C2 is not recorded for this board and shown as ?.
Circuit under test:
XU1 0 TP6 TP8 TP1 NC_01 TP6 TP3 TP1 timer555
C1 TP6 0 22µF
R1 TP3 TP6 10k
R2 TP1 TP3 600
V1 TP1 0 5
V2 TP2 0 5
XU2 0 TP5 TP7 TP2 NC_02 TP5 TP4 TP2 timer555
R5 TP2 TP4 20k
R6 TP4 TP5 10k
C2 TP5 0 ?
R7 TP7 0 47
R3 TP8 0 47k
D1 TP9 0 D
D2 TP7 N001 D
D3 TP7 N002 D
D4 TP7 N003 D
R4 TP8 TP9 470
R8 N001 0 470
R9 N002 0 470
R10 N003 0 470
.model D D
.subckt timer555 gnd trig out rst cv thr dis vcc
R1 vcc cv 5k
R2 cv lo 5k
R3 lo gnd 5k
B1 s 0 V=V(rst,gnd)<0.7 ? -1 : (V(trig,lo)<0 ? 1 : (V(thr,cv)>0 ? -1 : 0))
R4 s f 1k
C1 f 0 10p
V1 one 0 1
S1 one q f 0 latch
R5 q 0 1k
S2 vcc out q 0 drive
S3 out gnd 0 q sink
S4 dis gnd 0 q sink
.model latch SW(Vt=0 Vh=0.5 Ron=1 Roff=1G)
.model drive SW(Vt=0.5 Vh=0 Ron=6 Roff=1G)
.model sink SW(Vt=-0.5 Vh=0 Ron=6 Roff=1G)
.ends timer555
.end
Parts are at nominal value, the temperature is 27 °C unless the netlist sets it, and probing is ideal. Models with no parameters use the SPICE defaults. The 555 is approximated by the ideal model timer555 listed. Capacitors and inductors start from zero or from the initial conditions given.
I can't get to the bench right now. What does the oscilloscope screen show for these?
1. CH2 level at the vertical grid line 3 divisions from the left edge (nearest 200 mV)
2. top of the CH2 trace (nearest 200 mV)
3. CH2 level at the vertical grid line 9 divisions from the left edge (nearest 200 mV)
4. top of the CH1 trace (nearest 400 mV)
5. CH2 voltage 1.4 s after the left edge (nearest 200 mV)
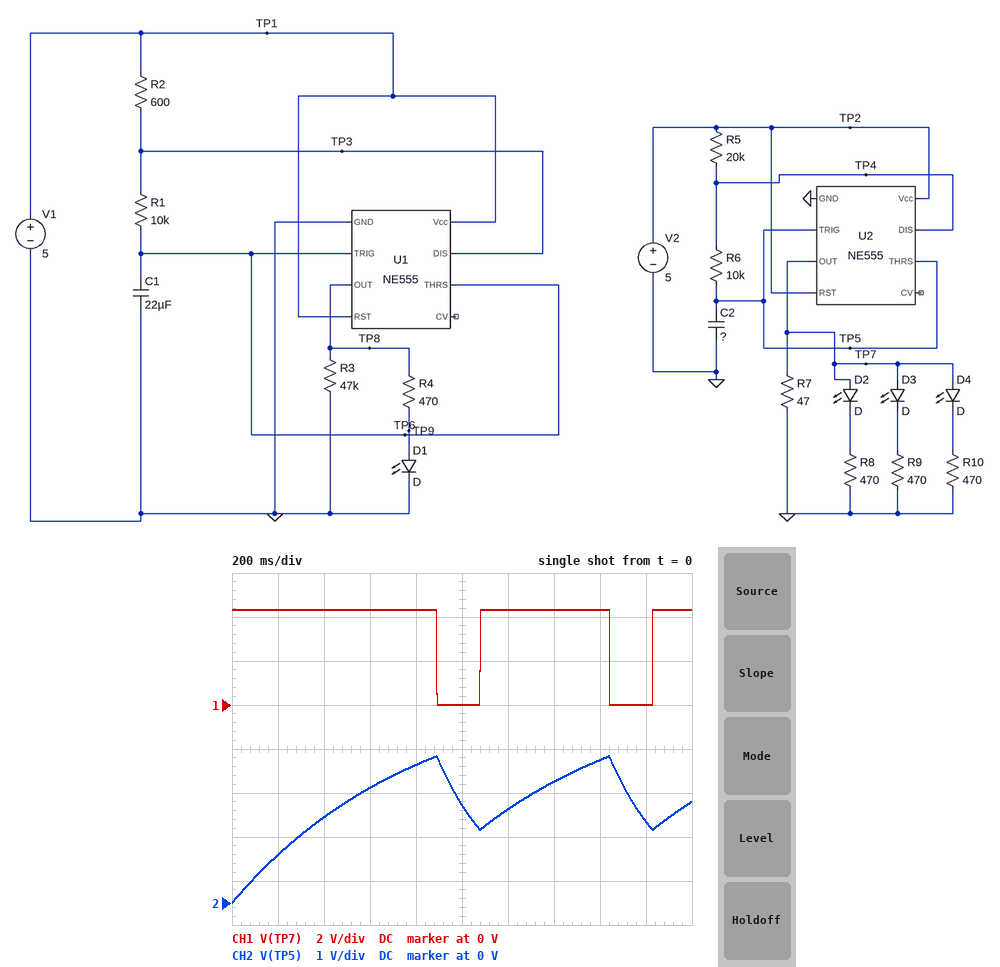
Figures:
2.6 V
3.4 V
1.8 V
4.4 V
2.8 V
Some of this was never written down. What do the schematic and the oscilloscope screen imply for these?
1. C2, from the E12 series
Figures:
27 µF
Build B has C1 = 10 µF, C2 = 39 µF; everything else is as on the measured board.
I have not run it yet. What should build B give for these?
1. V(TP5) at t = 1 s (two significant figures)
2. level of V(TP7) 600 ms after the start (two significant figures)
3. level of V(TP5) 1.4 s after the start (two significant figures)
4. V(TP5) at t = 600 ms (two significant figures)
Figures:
2.9 V
4.3 V
2.5 V
2.0 V
